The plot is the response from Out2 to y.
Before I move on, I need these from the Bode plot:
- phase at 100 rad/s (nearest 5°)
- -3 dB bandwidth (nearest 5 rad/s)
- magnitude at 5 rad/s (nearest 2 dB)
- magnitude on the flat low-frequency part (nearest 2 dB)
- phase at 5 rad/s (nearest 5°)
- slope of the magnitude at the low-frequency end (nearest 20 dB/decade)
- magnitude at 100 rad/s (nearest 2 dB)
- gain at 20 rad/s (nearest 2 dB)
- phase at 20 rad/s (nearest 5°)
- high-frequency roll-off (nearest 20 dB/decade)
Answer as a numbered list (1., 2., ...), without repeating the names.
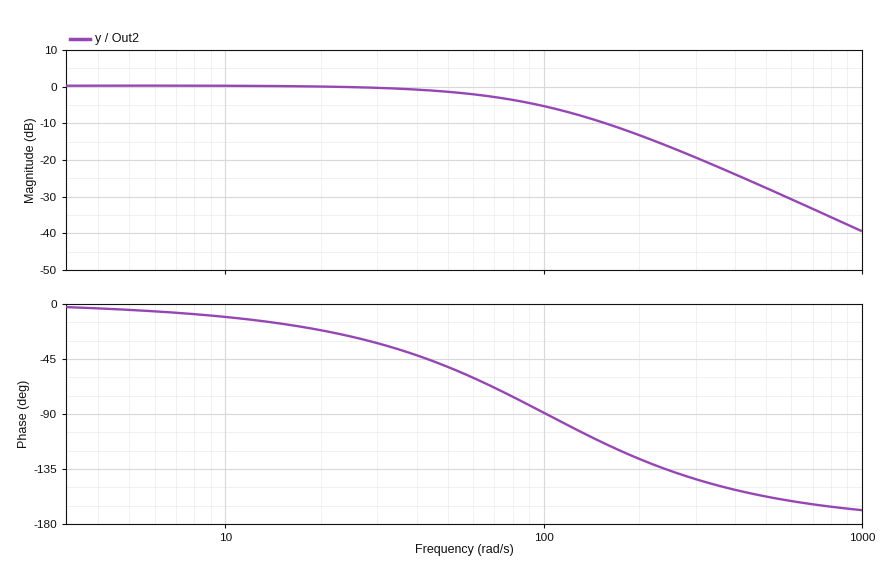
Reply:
1. -90°
2. 70 rad/s
3. 0 dB
4. 0 dB
5. -5°
6. 0 dB/decade
7. -6 dB
8. 0 dB
9. -20°
10. -40 dB/decade
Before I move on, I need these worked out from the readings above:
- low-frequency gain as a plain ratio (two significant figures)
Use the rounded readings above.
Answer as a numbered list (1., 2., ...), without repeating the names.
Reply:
1. 1.0
